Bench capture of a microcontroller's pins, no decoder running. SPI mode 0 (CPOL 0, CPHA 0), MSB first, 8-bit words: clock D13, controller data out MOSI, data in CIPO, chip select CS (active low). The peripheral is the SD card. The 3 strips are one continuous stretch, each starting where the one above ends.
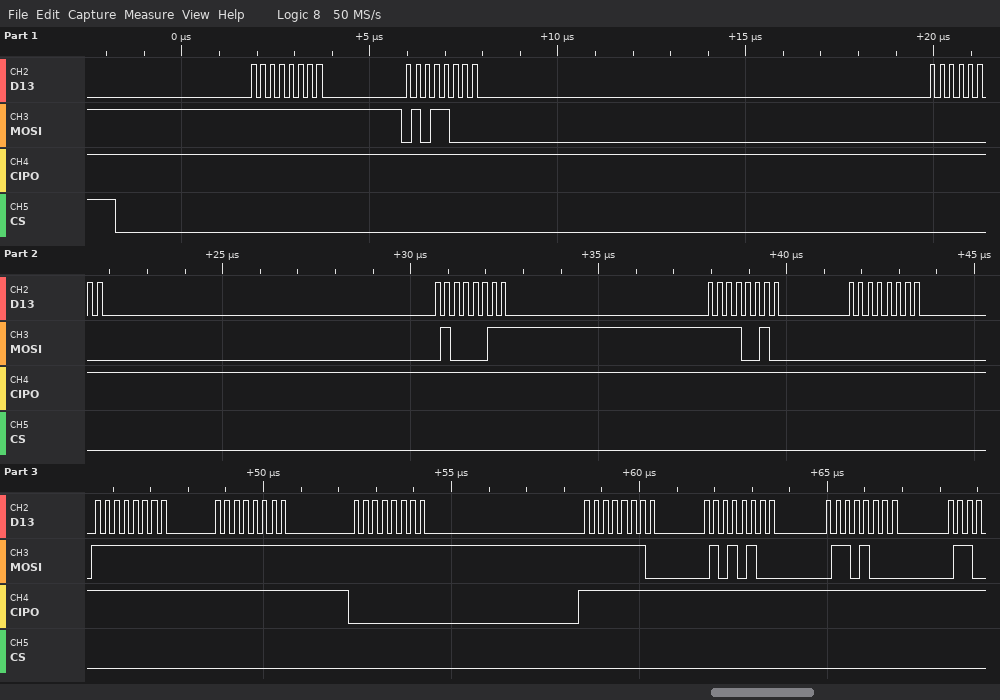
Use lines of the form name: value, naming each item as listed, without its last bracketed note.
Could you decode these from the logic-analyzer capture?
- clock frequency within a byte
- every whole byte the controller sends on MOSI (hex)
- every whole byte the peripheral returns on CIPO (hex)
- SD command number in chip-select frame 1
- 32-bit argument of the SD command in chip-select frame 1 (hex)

clock frequency within a byte: 4 MHz
every whole byte the controller sends on MOSI: 0xFF 0x58 0x00 0x43 0xF2 0x00 0xFF 0xFF 0xFF 0xFE 0x54 0x68
every whole byte the peripheral returns on CIPO: 0xFF 0xFF 0xFF 0xFF 0xFF 0xFF 0xFF 0xFF 0x00 0xFF 0xFF 0xFF
SD command number in chip-select frame 1: CMD24
32-bit argument of the SD command in chip-select frame 1: 0x0043F200
